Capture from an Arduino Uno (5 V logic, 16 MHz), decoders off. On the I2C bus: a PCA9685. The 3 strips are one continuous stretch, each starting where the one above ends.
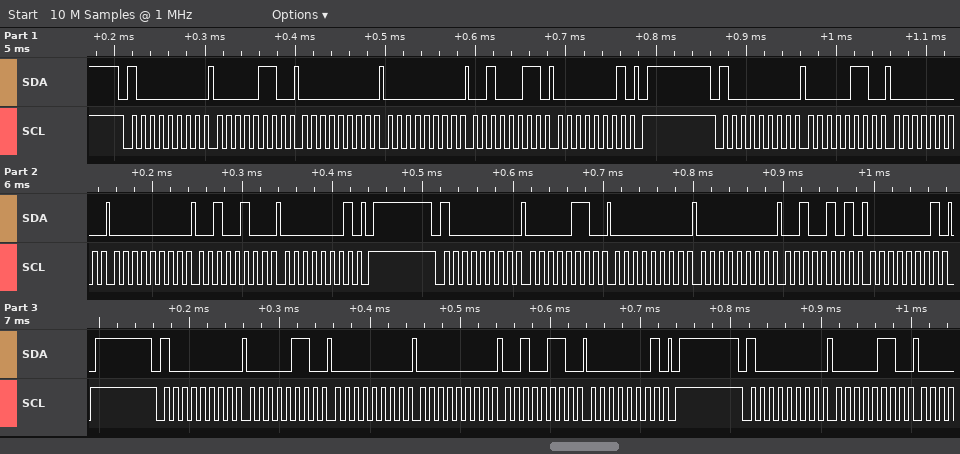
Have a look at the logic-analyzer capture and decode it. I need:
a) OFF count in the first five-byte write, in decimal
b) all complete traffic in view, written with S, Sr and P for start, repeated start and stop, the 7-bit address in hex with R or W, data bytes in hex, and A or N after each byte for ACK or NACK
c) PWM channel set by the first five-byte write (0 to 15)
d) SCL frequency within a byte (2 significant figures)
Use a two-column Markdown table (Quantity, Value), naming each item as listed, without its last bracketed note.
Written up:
| Quantity | Value |
|---|---|
| OFF count in the first five-byte write, in decimal | 291 |
| all complete traffic in view, written with S, Sr and P for start, repeated start and stop, the 7-bit address in hex with R or W, data bytes in hex, and A or N after each byte for ACK or NACK | S 40W A 06 A 00 A 00 A 23 A 01 A P S 40W A 06 A 00 A 00 A 24 A 01 A P S 40W A 06 A 00 A 00 A 25 A 01 A P S 40W A 06 A 00 A 00 A 26 A 01 A P S 40W A 06 A |
| PWM channel set by the first five-byte write | 0 |
| SCL frequency within a byte | 100 kHz |
